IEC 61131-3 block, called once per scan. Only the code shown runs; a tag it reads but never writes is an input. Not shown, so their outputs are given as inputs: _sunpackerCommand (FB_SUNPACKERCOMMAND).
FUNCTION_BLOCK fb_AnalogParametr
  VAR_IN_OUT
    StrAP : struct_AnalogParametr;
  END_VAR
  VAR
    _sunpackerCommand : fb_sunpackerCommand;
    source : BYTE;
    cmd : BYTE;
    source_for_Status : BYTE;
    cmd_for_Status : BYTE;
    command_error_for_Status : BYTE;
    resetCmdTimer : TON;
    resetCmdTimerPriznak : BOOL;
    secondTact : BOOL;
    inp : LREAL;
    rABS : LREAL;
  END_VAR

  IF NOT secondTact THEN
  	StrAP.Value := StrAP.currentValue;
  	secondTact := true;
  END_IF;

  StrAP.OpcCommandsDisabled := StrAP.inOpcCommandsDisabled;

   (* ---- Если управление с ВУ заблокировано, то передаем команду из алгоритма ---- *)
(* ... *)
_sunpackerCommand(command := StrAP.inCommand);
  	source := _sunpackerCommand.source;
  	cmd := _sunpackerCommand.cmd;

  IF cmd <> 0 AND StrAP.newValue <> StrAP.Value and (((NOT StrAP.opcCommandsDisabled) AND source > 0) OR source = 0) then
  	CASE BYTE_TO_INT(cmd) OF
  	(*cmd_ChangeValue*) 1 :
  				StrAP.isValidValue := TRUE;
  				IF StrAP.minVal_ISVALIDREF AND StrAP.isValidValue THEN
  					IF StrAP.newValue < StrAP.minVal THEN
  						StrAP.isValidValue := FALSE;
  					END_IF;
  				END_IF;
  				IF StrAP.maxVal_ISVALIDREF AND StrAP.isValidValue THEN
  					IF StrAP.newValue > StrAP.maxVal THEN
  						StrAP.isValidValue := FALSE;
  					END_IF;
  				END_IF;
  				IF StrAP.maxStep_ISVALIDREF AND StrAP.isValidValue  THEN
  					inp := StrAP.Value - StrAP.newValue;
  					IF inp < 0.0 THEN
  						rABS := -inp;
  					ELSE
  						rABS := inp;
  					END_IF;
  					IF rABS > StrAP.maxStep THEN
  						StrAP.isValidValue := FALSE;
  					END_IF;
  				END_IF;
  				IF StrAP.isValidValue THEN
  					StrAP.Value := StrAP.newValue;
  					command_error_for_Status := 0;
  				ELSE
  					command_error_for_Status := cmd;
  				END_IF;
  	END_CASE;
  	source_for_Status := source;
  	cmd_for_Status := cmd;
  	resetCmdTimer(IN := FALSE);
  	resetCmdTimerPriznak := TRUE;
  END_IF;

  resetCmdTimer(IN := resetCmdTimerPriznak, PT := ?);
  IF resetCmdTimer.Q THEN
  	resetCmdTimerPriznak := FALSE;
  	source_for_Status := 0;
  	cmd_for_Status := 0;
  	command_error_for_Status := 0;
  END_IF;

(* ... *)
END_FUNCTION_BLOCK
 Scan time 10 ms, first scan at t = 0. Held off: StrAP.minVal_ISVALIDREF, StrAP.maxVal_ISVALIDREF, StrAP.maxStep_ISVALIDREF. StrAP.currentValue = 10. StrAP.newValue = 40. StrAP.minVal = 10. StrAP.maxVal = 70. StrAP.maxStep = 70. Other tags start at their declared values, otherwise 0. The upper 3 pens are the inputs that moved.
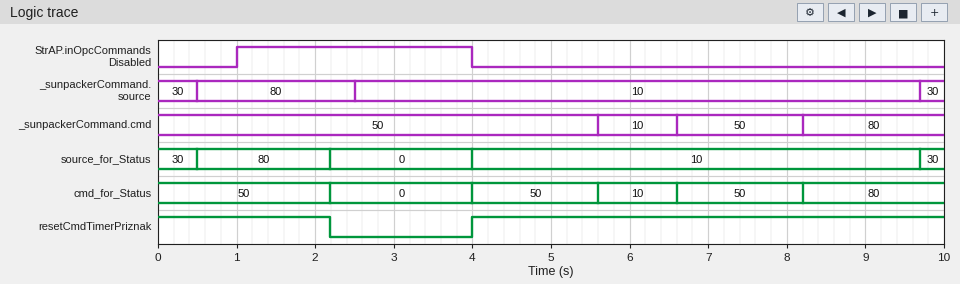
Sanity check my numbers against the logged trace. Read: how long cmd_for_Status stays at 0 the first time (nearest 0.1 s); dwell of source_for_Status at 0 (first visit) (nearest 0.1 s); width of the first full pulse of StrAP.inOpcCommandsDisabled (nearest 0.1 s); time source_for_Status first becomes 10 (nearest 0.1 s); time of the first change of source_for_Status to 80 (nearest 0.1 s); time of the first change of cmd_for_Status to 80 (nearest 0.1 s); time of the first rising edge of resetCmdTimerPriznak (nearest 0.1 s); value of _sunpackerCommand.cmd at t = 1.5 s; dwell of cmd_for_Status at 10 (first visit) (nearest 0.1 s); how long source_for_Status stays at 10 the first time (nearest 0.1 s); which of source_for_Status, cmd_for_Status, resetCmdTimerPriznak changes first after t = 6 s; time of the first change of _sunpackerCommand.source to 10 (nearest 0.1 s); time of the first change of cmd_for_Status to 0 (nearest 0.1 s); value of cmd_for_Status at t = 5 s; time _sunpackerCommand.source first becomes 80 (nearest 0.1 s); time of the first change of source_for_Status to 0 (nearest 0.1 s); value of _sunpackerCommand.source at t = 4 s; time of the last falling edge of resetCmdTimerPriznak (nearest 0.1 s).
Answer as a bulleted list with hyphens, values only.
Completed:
- 1.8 s
- 1.8 s
- 3.0 s
- 4.0 s
- 0.5 s
- 8.2 s
- 4.0 s
- 50
- 1.0 s
- 5.7 s
- cmd_for_Status
- 2.5 s
- 2.2 s
- 50
- 0.5 s
- 2.2 s
- 10
- 2.2 s
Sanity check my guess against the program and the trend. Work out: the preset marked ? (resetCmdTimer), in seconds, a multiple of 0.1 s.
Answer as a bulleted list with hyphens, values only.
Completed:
- 1.2 s
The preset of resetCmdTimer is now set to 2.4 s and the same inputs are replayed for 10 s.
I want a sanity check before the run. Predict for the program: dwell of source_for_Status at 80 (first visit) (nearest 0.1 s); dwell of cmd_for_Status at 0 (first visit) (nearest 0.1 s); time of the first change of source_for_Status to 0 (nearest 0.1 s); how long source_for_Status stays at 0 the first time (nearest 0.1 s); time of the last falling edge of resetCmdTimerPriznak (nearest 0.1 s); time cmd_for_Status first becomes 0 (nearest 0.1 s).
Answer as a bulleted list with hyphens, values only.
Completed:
- 2.9 s
- 0.6 s
- 3.4 s
- 0.6 s
- 3.4 s
- 3.4 s
